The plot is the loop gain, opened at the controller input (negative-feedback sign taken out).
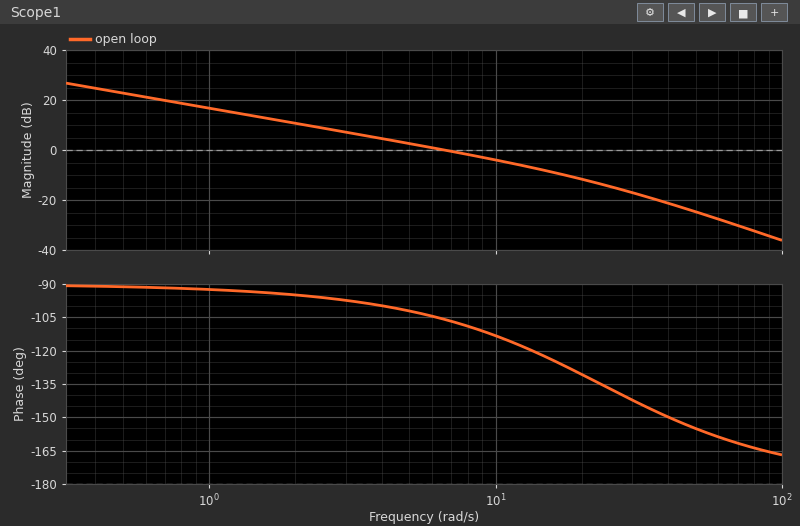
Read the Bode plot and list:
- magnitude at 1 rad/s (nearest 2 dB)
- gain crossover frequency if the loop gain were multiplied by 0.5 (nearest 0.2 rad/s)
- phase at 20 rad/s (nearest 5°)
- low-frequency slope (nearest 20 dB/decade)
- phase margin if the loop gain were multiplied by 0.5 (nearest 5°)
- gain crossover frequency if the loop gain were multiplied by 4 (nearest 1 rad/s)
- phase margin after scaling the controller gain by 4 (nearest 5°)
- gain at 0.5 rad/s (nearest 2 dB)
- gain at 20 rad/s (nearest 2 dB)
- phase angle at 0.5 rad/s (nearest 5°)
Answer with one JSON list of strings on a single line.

["16 dB", "3.4 rad/s", "-130°", "-20 dB/decade", "80°", "21 rad/s", "50°", "22 dB", "-12 dB", "-90°"]
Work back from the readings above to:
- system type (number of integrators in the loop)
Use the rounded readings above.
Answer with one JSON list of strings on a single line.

["1"]
